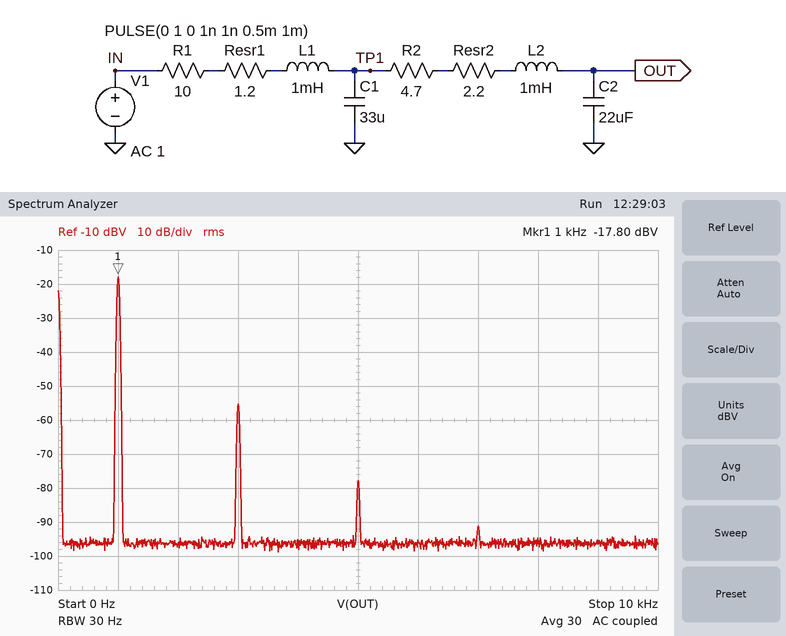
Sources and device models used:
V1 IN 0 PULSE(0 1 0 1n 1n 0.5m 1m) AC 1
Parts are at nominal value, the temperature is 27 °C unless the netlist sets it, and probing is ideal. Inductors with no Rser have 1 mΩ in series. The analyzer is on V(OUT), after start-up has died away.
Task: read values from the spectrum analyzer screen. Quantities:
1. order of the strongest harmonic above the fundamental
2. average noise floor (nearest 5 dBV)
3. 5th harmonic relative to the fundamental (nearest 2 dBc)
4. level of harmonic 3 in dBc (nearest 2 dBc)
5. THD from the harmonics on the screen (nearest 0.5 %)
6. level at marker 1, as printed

3
-95 dBV
-60 dBc
-38 dBc
1.5 %
-17.80 dBV
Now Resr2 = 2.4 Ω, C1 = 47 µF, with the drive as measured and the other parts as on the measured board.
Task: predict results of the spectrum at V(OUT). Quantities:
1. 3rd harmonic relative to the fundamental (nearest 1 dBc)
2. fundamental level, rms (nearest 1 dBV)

-39 dBc
-20 dBV
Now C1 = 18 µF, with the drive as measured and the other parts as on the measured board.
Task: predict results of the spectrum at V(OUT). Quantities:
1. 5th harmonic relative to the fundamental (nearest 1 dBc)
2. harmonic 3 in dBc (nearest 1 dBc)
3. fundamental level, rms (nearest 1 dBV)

-56 dBc
-33 dBc
-16 dBV
